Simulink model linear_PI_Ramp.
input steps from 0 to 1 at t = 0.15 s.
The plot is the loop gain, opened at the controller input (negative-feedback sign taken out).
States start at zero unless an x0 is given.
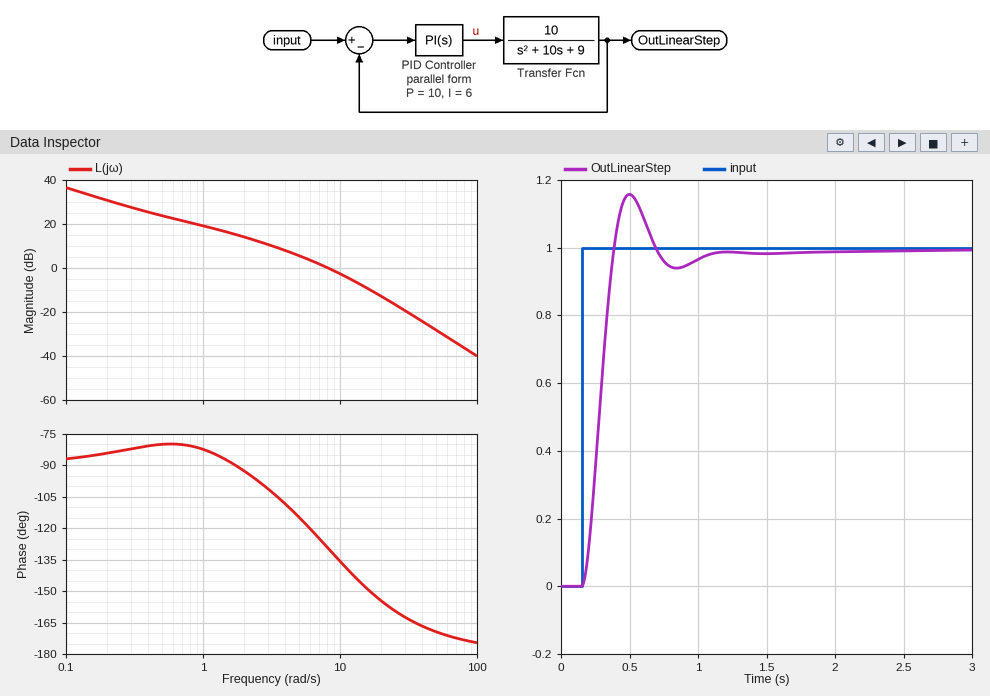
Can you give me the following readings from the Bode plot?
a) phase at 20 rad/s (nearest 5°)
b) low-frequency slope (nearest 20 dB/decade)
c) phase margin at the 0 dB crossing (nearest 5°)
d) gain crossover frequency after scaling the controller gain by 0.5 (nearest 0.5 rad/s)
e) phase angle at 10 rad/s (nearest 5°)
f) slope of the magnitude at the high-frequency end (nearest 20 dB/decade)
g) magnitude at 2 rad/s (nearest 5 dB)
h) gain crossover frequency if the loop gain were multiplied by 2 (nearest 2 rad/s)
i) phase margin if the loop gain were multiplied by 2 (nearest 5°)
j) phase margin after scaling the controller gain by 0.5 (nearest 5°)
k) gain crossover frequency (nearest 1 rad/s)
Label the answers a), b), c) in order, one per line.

a) -155°
b) -20 dB/decade
c) 50°
d) 5.0 rad/s
e) -135°
f) -40 dB/decade
g) 15 dB
h) 12 rad/s
i) 35°
j) 65°
k) 8 rad/s
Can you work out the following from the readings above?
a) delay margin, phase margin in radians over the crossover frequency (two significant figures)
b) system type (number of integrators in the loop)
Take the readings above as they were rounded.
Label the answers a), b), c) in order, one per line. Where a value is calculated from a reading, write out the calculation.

a) 50 × π / 180 / 8 = 0.11 s
b) 1
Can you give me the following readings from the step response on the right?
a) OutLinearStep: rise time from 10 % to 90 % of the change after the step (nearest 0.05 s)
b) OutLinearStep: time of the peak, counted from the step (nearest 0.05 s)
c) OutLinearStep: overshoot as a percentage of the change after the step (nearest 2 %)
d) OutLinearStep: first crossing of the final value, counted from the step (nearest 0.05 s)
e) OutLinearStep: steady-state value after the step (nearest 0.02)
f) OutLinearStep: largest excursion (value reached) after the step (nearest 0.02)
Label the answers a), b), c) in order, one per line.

a) 0.15 s
b) 0.35 s
c) 16 %
d) 0.25 s
e) 1.00
f) 1.16
